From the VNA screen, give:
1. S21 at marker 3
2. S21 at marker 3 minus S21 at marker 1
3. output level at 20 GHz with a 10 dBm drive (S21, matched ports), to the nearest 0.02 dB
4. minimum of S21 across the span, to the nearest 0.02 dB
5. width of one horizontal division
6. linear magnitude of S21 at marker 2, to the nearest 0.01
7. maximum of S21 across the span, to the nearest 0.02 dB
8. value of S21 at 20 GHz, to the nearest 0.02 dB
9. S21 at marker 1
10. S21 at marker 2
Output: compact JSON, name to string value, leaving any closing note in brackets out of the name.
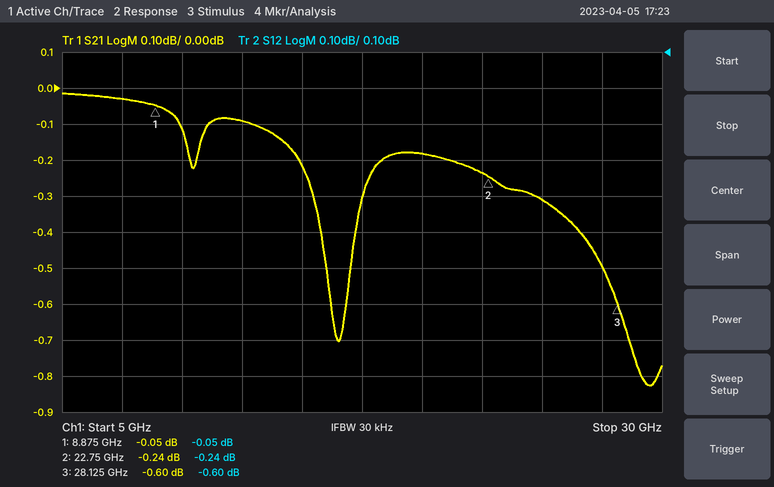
{"S21 at marker 3": "-0.60 dB", "S21 at marker 3 minus S21 at marker 1": "-0.55 dB", "output level at 20 GHz with a 10 dBm drive (S21, matched ports), to the nearest 0.02 dB": "9.82 dBm", "minimum of S21 across the span, to the nearest 0.02 dB": "-0.82 dB", "width of one horizontal division": "2.5 GHz", "linear magnitude of S21 at marker 2, to the nearest 0.01": "0.97", "maximum of S21 across the span, to the nearest 0.02 dB": "-0.02 dB", "value of S21 at 20 GHz, to the nearest 0.02 dB": "-0.18 dB", "S21 at marker 1": "-0.05 dB", "S21 at marker 2": "-0.24 dB"}
